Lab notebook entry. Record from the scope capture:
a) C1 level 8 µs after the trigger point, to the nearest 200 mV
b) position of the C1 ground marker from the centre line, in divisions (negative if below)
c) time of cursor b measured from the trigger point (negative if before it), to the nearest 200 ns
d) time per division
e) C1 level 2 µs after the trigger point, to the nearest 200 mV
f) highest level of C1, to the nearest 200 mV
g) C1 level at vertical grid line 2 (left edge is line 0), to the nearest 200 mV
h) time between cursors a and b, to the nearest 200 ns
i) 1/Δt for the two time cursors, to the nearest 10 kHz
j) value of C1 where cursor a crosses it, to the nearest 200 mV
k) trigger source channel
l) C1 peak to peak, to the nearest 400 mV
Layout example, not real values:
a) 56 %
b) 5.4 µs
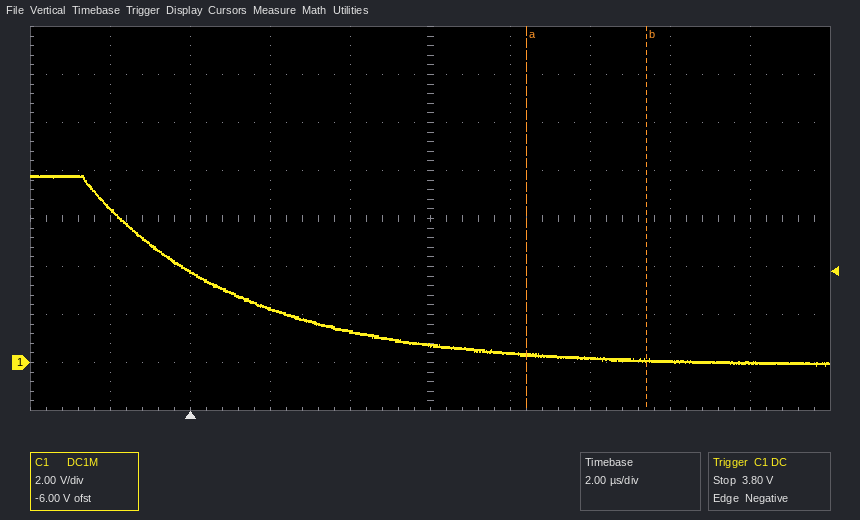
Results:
a) 400 mV
b) -3.0 div
c) +11.4 µs
d) 2 µs
e) 2.2 V
f) 7.8 V
g) 3.8 V
h) 3.0 µs
i) 330 kHz
j) 400 mV
k) C1
l) 8.0 V
